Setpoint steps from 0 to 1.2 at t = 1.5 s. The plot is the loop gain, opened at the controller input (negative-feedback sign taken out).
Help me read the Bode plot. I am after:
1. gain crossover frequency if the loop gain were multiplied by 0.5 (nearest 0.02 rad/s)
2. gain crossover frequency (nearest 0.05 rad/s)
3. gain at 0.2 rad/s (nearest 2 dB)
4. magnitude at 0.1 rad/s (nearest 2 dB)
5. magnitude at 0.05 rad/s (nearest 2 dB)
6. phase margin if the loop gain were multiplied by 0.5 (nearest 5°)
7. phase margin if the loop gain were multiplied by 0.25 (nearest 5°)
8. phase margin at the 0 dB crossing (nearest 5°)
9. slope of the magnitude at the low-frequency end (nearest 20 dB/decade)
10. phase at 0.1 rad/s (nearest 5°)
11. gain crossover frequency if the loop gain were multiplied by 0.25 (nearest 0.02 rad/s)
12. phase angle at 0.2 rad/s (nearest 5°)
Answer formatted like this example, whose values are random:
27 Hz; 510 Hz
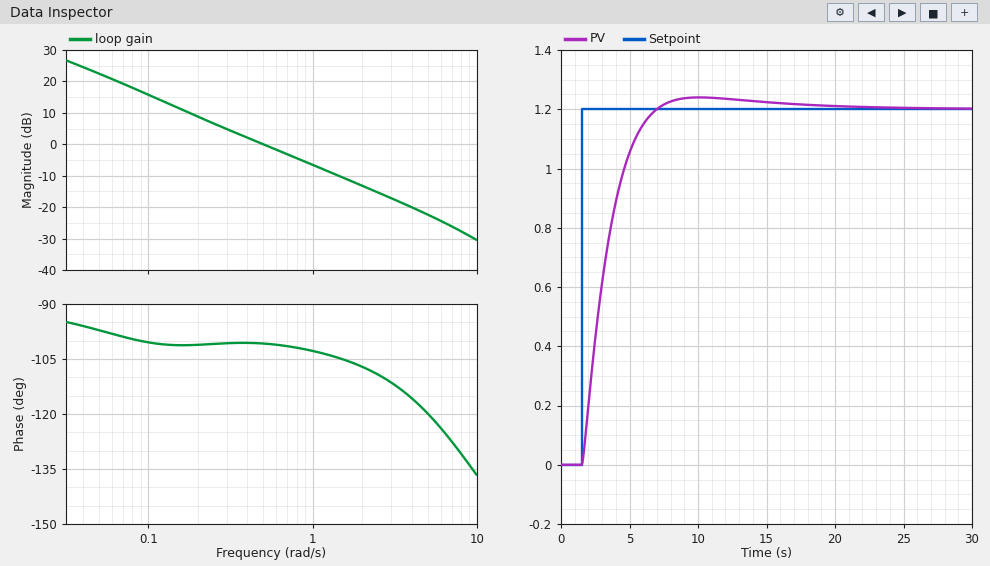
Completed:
0.26 rad/s; 0.50 rad/s; 8 dB; 16 dB; 22 dB; 80°; 80°; 80°; -20 dB/decade; -100°; 0.14 rad/s; -100°
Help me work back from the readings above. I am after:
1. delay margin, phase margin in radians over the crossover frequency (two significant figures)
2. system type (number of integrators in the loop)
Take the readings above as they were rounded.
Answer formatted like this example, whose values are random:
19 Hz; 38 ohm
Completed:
2.8 s; 1
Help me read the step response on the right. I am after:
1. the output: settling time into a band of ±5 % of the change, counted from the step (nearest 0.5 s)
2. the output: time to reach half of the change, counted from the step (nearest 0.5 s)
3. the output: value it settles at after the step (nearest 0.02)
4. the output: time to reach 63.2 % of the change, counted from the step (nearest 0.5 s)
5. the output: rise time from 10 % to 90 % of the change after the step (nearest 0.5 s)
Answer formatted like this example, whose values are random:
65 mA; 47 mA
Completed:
4.5 s; 1.5 s; 1.20; 2.0 s; 3.5 s
